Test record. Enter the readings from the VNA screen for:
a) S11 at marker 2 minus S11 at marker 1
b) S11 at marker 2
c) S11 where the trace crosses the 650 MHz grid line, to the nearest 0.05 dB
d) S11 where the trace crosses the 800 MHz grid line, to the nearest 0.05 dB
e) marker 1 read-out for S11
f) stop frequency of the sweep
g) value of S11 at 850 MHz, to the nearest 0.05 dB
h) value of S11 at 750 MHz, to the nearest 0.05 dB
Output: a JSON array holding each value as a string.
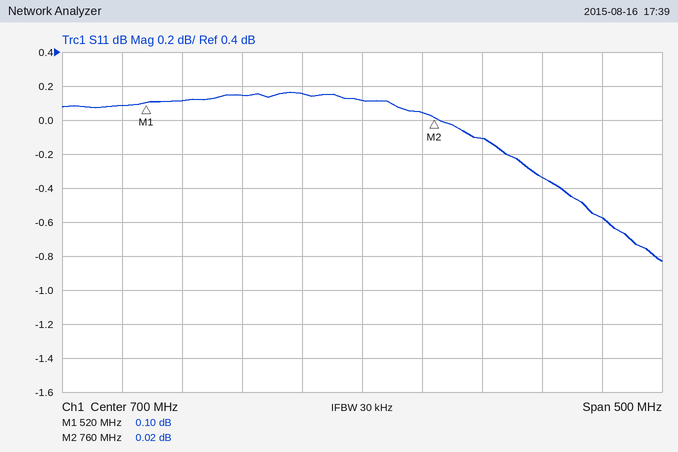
["-0.08 dB", "0.02 dB", "0.15 dB", "-0.10 dB", "0.10 dB", "950 MHz", "-0.35 dB", "0.05 dB"]
